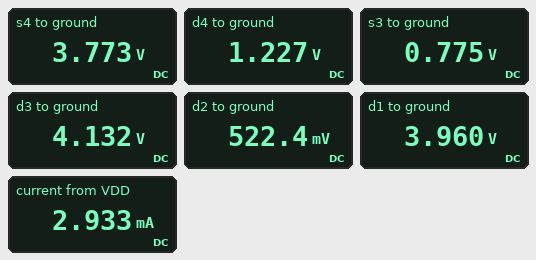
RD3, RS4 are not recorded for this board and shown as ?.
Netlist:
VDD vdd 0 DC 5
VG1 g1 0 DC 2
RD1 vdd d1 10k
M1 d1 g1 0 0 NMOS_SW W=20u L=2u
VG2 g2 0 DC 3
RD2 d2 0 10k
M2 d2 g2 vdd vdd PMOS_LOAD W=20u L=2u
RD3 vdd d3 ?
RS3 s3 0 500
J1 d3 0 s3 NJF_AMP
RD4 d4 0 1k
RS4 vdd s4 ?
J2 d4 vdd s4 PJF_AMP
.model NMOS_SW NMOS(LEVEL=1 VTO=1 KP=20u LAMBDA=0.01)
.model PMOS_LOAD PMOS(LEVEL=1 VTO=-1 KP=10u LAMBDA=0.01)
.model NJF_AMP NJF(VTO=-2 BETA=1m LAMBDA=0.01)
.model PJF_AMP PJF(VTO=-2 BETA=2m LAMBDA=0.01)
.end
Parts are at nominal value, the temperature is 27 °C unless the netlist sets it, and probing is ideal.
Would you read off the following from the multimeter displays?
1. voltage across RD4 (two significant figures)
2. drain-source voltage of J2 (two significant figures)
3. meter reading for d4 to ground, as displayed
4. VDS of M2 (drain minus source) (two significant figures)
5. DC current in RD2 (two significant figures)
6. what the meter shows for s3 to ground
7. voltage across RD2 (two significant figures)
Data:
1.2 V
-2.5 V
1.227 V
-4.5 V
52 µA
0.775 V
520 mV
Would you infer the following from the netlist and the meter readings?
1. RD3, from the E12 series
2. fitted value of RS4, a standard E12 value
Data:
560 Ω
1 kΩ
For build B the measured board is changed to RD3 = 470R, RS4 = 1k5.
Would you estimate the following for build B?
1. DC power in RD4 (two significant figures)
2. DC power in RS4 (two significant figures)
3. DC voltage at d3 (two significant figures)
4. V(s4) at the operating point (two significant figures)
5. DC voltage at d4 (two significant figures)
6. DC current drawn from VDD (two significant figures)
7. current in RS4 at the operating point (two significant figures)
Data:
800 µW
1.2 mW
4.3 V
3.7 V
890 mV
2.6 mA
890 µA
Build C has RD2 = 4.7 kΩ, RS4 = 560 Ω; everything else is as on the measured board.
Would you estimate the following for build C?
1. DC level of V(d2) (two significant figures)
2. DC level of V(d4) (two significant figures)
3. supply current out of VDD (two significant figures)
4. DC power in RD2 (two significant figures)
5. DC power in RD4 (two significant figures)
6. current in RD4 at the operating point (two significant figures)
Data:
250 mV
1.9 V
3.6 mA
13 µW
3.5 mW
1.9 mA
